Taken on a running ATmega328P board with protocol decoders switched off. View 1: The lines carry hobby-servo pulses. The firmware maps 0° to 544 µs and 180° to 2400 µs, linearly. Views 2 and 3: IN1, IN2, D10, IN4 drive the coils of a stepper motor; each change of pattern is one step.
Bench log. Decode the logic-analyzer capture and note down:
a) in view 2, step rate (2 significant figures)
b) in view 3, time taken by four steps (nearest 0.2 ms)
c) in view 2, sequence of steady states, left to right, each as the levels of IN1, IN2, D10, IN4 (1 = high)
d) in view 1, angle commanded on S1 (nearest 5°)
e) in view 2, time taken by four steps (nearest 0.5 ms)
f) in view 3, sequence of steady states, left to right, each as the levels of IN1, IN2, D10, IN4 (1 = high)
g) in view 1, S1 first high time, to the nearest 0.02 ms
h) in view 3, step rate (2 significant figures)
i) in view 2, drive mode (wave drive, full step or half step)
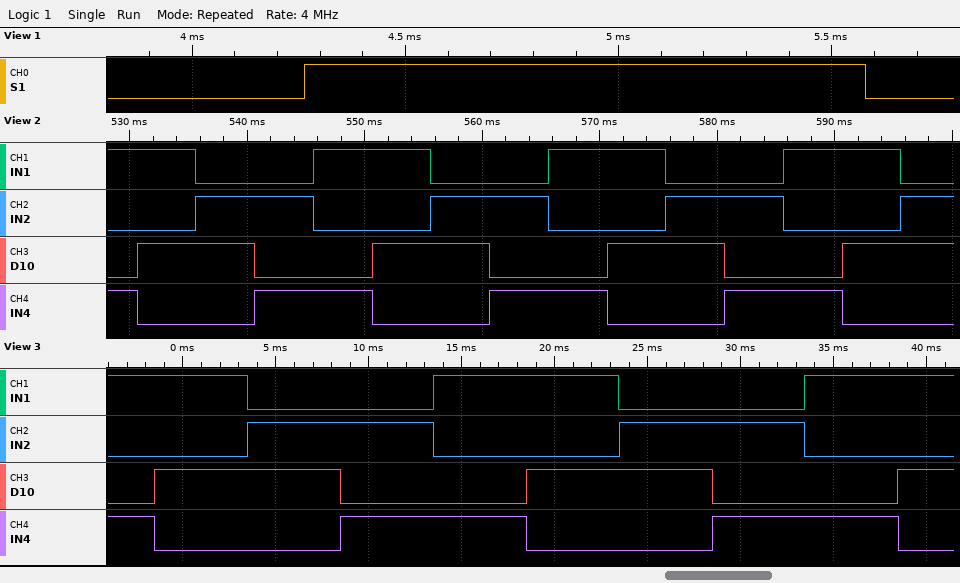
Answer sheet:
200 steps/s
20.0 ms
1001 1010 0110 0101 1001 1010 0110 0101 1001 1010 0110 0101 1001 1010 0110
75°
20.0 ms
1001 1010 0110 0101 1001 1010 0110 0101 1001 1010
1.32 ms
200 steps/s
full step
